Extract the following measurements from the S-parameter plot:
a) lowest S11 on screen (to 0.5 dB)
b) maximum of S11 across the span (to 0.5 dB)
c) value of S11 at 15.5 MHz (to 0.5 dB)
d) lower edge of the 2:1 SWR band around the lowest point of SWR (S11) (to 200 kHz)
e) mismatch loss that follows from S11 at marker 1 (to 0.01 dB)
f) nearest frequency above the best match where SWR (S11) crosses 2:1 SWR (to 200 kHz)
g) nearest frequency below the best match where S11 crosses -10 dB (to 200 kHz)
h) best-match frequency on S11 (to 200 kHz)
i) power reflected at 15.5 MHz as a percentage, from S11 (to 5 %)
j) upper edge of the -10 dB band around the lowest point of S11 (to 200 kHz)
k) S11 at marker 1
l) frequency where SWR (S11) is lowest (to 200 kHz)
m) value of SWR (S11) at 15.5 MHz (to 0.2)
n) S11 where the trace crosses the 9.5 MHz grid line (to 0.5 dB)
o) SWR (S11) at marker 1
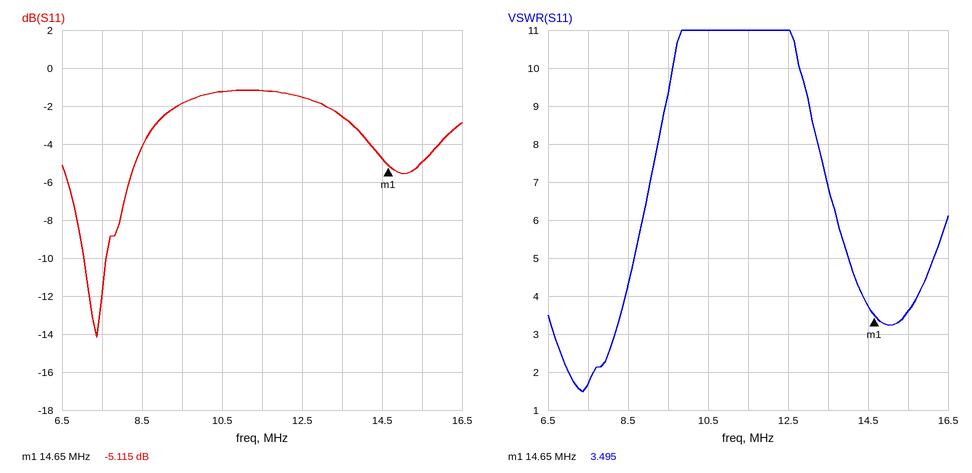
-14.0 dB
-1.0 dB
-5.0 dB
7.0 MHz
1.60 dB
7.6 MHz
7.0 MHz
7.4 MHz
30 %
7.6 MHz
-5.115 dB
7.4 MHz
3.6
-2.0 dB
3.495
